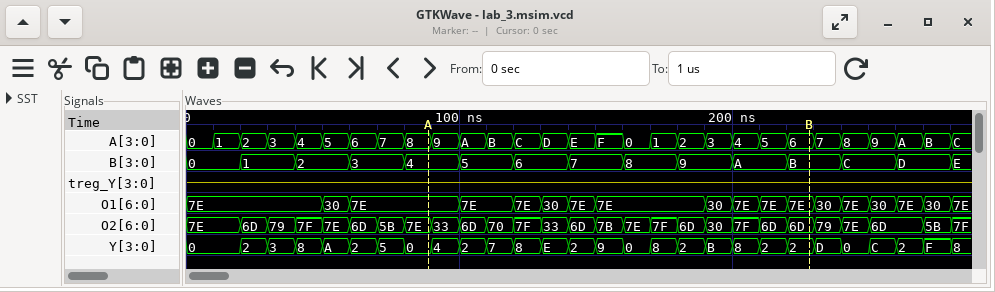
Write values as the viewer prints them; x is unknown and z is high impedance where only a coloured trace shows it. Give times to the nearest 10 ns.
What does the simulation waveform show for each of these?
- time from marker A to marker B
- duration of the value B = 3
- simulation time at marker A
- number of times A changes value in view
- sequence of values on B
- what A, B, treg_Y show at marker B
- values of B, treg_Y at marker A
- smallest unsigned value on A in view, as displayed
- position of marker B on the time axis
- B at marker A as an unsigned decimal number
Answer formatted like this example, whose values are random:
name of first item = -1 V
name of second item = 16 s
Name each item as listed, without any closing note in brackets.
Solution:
time from marker A to marker B = 140 ns
duration of the value B = 3 = 20 ns
simulation time at marker A = 90 ns
number of times A changes value in view = 28
sequence of values on B = 0, 1, 2, 3, 4, 5, 6, 7, 8, 9, A, B, C, D, E
what A, B, treg_Y show at marker B = A=6, B=B, treg_Y=z
values of B, treg_Y at marker A = B=4, treg_Y=z
smallest unsigned value on A in view, as displayed = 0
position of marker B on the time axis = 230 ns
B at marker A as an unsigned decimal number = 4
